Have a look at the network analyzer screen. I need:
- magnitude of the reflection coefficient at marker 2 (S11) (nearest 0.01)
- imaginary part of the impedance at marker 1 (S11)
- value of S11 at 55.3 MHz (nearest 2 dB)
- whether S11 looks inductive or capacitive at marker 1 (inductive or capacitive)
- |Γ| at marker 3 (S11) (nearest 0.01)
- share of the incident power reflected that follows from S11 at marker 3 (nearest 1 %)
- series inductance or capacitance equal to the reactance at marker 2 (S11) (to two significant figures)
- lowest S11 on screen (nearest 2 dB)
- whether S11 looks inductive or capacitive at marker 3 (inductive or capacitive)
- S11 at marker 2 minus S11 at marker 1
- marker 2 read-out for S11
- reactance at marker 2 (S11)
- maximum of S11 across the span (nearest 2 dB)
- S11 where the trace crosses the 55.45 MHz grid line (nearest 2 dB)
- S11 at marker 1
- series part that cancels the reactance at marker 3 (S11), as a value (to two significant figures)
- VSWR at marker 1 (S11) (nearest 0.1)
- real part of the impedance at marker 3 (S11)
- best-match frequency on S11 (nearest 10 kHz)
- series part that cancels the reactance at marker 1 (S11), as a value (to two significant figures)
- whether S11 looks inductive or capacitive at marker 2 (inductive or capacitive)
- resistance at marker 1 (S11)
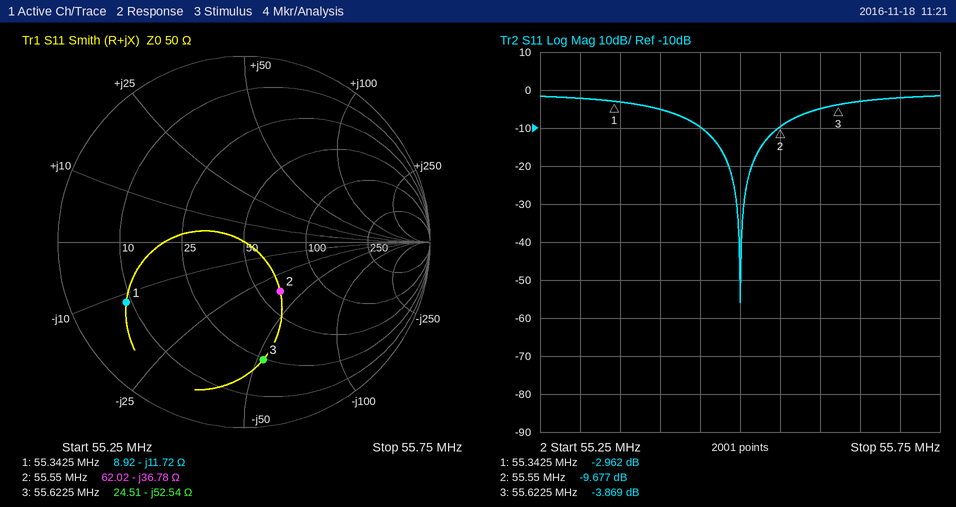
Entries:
0.33
-11.72 Ω
-2 dB
capacitive
0.64
41 %
78 pF
-56 dB
capacitive
-6.715 dB
-9.677 dB
-36.78 Ω
-2 dB
-10 dB
-2.962 dB
150 nH
5.9
24.51 Ω
55.50 MHz
34 nH
capacitive
8.92 Ω
